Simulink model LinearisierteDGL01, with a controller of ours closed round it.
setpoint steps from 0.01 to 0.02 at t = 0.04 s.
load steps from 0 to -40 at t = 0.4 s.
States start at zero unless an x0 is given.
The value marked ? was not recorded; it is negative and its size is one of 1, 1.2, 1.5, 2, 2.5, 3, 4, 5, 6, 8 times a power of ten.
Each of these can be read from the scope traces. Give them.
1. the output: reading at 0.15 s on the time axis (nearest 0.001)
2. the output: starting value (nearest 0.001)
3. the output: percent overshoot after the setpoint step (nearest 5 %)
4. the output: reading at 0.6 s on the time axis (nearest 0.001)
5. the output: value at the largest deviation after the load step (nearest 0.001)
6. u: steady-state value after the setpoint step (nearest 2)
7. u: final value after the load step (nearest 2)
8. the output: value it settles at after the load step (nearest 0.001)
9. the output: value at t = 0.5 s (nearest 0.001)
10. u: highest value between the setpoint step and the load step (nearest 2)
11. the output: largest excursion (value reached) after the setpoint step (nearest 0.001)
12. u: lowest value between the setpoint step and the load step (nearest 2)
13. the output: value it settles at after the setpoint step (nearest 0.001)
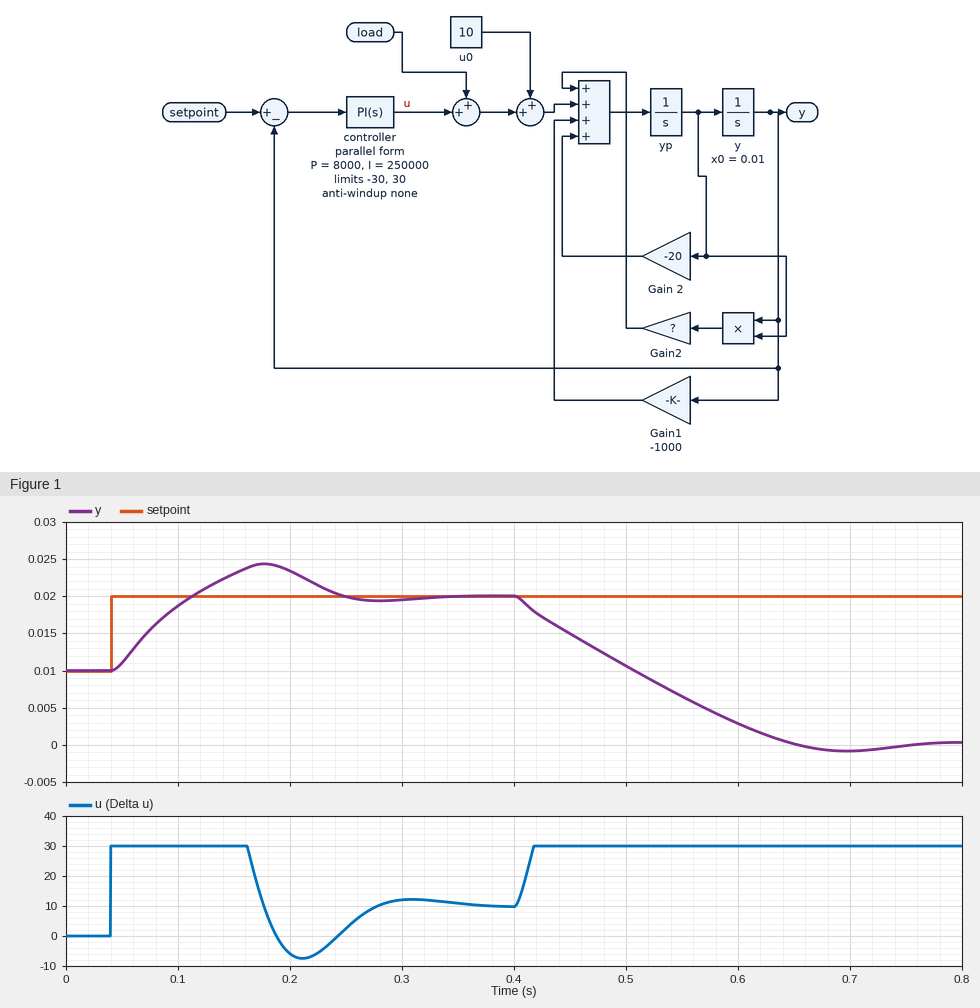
0.023
0.010
45 %
0.003
-0.001
10
30
0.000
0.011
30
0.024
-8
0.020
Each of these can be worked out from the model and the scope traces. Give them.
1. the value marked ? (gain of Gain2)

-10000
